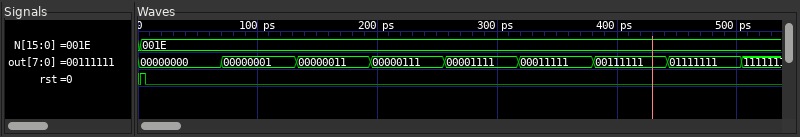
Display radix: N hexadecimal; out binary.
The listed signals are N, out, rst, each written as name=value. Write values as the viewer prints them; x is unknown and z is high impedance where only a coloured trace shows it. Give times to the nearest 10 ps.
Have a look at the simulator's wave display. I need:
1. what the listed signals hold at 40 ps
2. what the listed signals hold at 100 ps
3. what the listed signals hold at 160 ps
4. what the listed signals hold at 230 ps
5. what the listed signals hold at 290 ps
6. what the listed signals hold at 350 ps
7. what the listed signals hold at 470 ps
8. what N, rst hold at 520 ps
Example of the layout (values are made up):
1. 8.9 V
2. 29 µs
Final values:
1. N=001E, out=00000000, rst=0
2. N=001E, out=00000001, rst=0
3. N=001E, out=00000011, rst=0
4. N=001E, out=00000111, rst=0
5. N=001E, out=00001111, rst=0
6. N=001E, out=00011111, rst=0
7. N=001E, out=01111111, rst=0
8. N=001E, rst=0
